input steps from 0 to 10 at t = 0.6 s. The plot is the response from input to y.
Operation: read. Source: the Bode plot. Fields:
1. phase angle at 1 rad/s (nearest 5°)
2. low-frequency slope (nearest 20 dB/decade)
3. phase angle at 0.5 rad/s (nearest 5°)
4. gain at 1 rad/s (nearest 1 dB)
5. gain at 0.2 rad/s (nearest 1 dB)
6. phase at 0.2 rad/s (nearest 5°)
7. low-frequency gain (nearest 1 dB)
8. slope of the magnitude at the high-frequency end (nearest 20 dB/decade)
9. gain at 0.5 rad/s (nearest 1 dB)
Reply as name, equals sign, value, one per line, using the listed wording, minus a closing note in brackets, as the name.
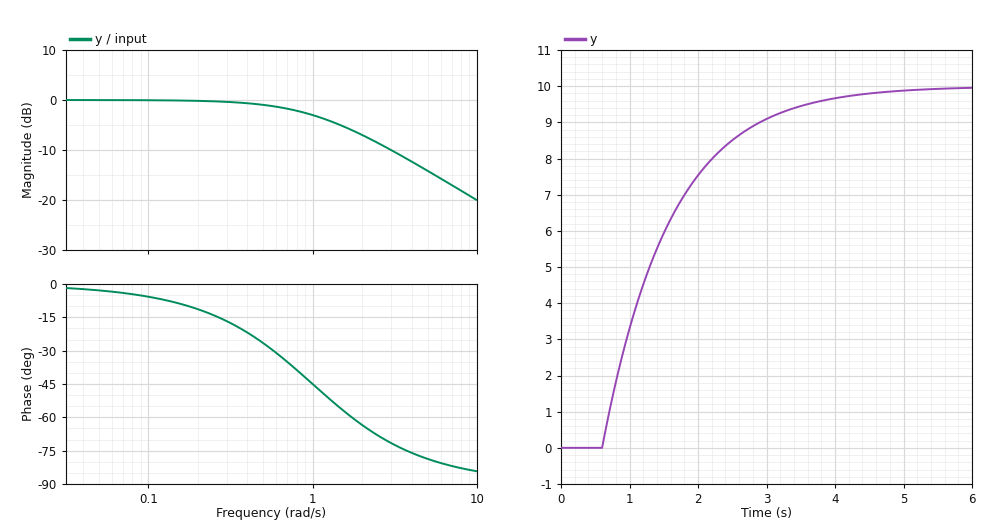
phase angle at 1 rad/s = -45°
low-frequency slope = 0 dB/decade
phase angle at 0.5 rad/s = -25°
gain at 1 rad/s = -3 dB
gain at 0.2 rad/s = 0 dB
phase at 0.2 rad/s = -10°
low-frequency gain = 0 dB
slope of the magnitude at the high-frequency end = -20 dB/decade
gain at 0.5 rad/s = -1 dB
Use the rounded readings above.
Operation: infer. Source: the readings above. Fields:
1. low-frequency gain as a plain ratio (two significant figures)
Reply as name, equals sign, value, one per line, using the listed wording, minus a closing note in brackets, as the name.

low-frequency gain as a plain ratio = 1.0
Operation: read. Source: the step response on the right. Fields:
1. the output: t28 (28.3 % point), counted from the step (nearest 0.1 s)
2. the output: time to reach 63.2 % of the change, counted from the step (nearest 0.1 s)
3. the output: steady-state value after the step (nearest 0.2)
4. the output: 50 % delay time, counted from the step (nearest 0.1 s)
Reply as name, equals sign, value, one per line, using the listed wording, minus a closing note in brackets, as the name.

the output: t28 (28.3 % point), counted from the step = 0.3 s
the output: time to reach 63.2 % of the change, counted from the step = 1.0 s
the output: steady-state value after the step = 10.0
the output: 50 % delay time, counted from the step = 0.7 s
